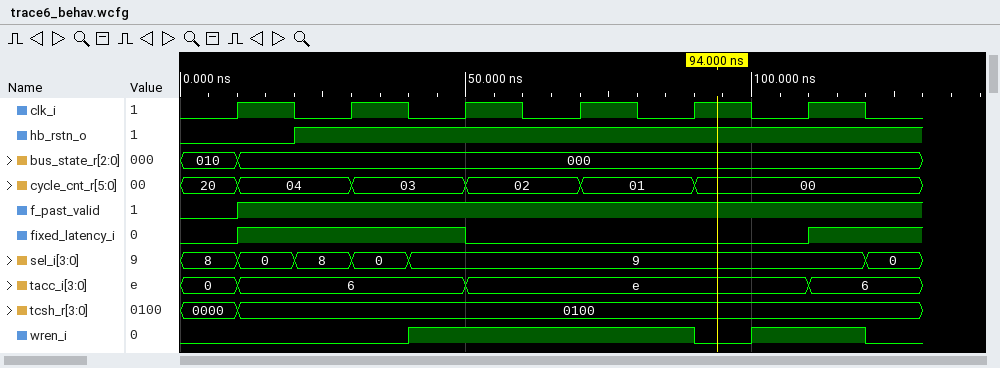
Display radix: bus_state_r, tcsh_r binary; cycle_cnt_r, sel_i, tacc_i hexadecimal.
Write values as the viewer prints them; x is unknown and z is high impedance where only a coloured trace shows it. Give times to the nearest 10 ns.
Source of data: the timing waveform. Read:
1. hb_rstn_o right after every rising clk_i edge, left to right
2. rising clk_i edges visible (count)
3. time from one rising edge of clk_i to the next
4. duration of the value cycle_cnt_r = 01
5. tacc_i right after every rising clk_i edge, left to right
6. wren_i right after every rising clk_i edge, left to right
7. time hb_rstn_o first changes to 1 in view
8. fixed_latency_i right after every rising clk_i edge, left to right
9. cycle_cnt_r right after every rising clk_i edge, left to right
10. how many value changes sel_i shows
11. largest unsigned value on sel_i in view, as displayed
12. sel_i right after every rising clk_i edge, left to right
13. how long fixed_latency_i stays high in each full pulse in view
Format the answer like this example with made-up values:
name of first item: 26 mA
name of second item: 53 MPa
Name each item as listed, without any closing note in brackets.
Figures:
hb_rstn_o right after every rising clk_i edge, left to right: 0 1 1 1 1 1
rising clk_i edges visible: 6
time from one rising edge of clk_i to the next: 20 ns
duration of the value cycle_cnt_r = 01: 20 ns
tacc_i right after every rising clk_i edge, left to right: 6, 6, e, e, e, 6
wren_i right after every rising clk_i edge, left to right: 0 0 1 1 0 1
time hb_rstn_o first changes to 1 in view: 20 ns
fixed_latency_i right after every rising clk_i edge, left to right: 1 1 0 0 0 1
cycle_cnt_r right after every rising clk_i edge, left to right: 04, 03, 02, 01, 00, 00
how many value changes sel_i shows: 5
largest unsigned value on sel_i in view, as displayed: 9
sel_i right after every rising clk_i edge, left to right: 0, 0, 9, 9, 9, 9
how long fixed_latency_i stays high in each full pulse in view: 40 ns
